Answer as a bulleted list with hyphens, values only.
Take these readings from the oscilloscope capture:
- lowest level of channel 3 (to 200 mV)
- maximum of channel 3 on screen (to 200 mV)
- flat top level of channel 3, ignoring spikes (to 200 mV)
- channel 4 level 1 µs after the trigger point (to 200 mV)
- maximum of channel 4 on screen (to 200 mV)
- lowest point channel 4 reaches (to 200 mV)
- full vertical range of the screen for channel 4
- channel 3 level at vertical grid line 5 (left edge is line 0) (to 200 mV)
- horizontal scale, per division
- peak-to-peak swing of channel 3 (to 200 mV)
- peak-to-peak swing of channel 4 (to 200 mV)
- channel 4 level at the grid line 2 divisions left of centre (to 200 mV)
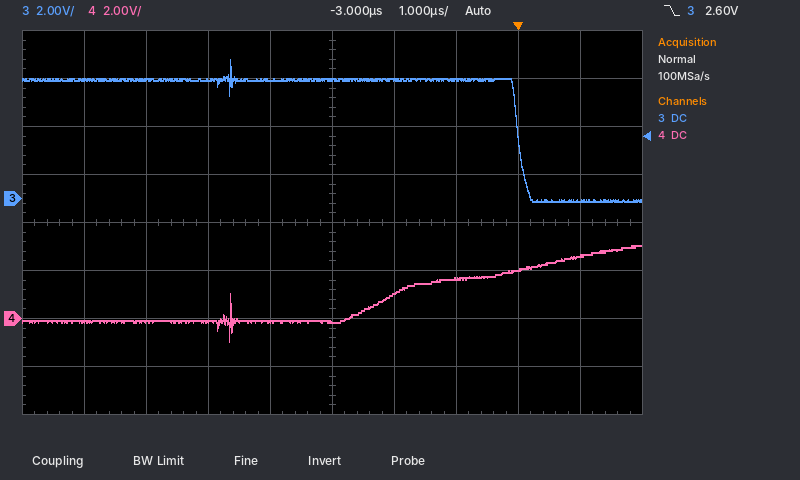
- -200 mV
- 5.8 V
- 5.0 V
- 2.6 V
- 3.0 V
- -1.0 V
- 16 V
- 5.0 V
- 1 µs
- 6.0 V
- 4.0 V
- -200 mV
